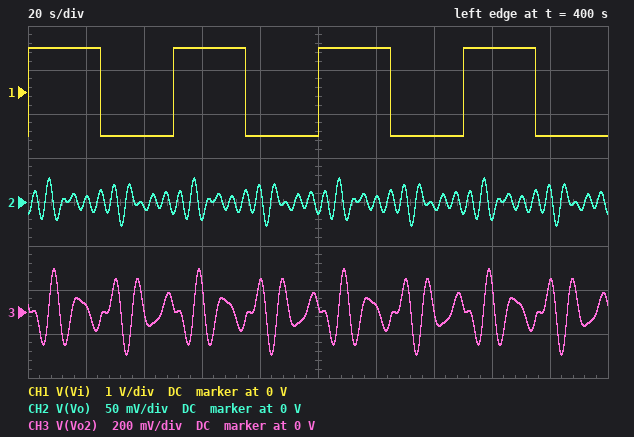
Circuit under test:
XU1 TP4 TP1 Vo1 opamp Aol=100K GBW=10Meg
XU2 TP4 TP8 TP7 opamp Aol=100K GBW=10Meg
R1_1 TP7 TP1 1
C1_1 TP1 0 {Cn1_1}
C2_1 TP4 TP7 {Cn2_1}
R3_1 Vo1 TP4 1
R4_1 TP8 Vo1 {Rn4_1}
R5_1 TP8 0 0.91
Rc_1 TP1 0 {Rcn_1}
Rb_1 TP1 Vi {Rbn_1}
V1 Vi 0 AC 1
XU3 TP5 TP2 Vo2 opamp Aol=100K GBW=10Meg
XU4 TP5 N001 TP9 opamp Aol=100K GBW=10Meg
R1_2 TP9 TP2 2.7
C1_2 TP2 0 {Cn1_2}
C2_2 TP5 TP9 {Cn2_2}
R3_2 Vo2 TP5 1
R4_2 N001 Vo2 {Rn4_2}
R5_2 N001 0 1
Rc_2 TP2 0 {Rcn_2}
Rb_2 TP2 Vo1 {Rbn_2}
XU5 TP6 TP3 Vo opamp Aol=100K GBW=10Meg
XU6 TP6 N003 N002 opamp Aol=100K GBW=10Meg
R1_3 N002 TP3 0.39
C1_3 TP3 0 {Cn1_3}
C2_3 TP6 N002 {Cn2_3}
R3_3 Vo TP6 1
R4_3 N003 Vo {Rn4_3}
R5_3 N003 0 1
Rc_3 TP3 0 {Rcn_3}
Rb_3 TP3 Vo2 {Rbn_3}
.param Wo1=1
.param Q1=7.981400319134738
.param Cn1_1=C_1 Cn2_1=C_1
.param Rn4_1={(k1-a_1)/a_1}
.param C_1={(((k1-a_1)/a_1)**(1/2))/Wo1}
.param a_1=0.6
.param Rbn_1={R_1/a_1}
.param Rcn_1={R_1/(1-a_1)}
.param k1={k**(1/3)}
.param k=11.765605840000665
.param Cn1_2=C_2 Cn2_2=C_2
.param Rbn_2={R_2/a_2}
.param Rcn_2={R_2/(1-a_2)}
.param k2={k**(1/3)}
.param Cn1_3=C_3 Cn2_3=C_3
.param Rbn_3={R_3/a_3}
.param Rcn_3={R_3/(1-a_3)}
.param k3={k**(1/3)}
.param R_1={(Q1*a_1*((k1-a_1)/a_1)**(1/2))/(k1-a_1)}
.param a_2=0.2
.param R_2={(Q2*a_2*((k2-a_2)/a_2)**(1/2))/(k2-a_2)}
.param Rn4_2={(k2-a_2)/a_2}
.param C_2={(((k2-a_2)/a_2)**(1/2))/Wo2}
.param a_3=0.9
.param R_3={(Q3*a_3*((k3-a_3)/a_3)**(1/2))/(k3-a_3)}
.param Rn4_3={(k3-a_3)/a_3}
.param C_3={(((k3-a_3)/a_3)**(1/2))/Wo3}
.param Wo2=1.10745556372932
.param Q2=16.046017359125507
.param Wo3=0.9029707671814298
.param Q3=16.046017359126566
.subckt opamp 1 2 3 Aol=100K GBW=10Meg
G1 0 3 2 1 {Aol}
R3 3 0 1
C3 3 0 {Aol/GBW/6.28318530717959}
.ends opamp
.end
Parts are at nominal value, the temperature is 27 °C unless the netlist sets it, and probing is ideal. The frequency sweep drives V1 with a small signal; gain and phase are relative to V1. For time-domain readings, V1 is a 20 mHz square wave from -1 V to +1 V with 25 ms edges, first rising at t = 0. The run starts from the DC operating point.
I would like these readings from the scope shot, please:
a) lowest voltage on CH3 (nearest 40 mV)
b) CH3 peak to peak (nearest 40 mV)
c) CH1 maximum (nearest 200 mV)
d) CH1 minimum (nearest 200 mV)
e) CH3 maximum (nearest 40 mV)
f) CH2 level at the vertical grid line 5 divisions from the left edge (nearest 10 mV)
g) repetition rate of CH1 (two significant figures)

-200 mV
400 mV
1.0 V
-1.0 V
200 mV
-10 mV
20 mHz
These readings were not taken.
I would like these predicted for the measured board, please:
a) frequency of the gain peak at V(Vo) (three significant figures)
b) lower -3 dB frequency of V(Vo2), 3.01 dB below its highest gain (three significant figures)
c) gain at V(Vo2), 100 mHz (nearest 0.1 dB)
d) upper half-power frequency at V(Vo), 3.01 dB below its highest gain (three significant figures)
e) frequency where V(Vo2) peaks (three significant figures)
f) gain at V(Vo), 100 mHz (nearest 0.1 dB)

230 mHz
103 mHz
-8.8 dB
234 mHz
108 mHz
-35.3 dB
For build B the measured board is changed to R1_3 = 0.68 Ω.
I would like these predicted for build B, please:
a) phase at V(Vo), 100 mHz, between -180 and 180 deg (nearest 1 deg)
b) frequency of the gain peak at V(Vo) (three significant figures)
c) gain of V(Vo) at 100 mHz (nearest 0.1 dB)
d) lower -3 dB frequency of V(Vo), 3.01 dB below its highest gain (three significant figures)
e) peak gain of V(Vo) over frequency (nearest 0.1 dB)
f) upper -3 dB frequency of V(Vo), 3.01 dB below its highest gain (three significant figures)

-135 deg
173 mHz
-28.8 dB
167 mHz
0.5 dB
177 mHz
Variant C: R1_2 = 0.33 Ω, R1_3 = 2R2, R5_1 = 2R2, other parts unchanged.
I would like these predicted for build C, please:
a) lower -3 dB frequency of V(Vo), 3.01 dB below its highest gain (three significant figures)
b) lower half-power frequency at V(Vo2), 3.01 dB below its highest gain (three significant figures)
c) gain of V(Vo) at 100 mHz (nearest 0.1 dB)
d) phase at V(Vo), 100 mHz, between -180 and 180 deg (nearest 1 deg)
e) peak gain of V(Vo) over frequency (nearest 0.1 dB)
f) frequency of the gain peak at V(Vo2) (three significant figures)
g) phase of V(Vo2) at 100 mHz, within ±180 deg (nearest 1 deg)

94.5 mHz
301 mHz
-24.4 dB
92 deg
-24.1 dB
307 mHz
126 deg
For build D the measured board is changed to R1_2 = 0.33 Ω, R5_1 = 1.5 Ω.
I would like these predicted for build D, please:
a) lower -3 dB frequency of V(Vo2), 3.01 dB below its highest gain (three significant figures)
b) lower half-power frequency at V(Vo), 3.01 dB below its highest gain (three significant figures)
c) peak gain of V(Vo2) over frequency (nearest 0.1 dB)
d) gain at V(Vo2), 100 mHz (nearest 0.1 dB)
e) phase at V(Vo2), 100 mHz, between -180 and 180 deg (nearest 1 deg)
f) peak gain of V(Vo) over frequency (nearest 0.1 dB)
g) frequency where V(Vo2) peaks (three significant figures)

301 mHz
226 mHz
-10.3 dB
-37.0 dB
163 deg
-23.3 dB
307 mHz
